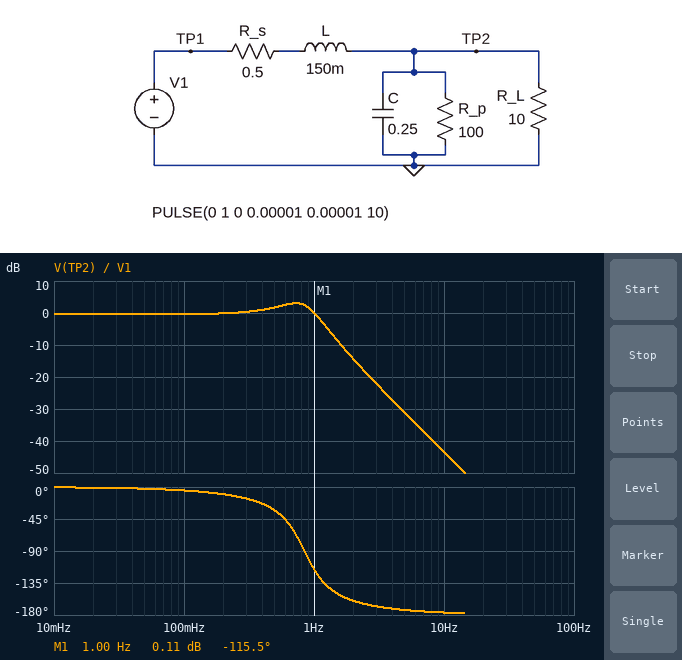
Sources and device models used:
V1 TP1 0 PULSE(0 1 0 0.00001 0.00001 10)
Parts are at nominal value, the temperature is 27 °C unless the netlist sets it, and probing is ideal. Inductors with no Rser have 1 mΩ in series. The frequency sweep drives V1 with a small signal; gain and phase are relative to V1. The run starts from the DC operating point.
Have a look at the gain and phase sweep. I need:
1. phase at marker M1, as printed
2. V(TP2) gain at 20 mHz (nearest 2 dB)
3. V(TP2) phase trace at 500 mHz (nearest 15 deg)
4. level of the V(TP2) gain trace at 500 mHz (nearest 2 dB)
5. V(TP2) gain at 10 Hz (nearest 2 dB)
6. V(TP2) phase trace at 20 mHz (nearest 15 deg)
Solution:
-115.5 deg
0 dB
-30 deg
2 dB
-44 dB
0 deg
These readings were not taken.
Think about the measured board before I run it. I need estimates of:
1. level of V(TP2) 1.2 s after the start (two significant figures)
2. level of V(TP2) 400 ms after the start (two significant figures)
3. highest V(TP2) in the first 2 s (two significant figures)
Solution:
870 mV
970 mV
1.2 V
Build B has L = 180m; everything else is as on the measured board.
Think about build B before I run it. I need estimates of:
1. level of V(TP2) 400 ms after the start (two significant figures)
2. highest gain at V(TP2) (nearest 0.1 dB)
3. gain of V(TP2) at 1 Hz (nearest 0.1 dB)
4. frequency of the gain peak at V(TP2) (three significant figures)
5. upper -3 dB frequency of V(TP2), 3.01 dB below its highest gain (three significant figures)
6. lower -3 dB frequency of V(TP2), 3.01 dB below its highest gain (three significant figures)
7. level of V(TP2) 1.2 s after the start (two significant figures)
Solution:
900 mV
3.6 dB
-1.3 dB
680 mHz
914 mHz
299 mHz
890 mV
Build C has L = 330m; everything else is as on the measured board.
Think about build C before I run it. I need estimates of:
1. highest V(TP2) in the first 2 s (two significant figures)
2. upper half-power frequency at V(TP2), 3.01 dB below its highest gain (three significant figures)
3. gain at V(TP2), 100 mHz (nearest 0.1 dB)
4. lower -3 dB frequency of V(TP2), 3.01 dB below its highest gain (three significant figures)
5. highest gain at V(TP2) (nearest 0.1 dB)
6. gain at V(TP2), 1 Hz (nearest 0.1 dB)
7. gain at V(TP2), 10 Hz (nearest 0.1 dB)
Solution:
1.3 V
668 mHz
-0.2 dB
324 mHz
5.1 dB
-7.7 dB
-50.2 dB
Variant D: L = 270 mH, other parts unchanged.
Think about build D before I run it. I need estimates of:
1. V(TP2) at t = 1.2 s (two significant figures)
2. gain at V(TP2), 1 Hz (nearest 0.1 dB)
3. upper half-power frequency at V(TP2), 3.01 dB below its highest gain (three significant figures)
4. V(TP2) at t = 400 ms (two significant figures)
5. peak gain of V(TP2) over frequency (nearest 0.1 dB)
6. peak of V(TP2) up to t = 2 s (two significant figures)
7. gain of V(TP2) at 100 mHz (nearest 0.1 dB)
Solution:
1.1 V
-5.5 dB
741 mHz
730 mV
4.6 dB
1.3 V
-0.3 dB
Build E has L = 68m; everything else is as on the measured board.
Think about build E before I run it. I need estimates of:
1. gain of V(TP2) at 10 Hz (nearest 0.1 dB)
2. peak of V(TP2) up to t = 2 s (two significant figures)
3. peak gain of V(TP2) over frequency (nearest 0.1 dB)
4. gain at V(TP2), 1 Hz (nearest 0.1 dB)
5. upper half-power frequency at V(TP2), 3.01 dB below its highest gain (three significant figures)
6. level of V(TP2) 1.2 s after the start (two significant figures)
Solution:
-36.5 dB
1.1 V
0.8 dB
0.7 dB
1.47 Hz
950 mV
